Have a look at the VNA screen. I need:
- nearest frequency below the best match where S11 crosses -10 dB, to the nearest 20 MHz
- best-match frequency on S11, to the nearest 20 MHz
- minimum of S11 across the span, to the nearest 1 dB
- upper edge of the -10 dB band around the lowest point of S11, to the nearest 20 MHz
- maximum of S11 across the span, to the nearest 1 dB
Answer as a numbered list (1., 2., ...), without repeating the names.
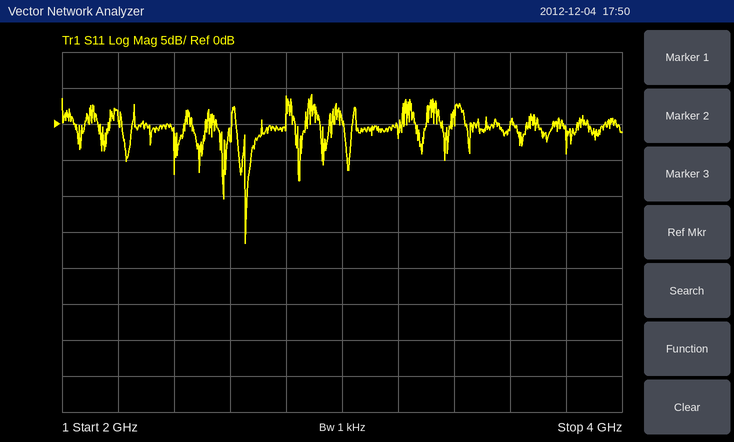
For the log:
1. 2.66 GHz
2. 2.66 GHz
3. -17 dB
4. 2.66 GHz
5. 4 dB
